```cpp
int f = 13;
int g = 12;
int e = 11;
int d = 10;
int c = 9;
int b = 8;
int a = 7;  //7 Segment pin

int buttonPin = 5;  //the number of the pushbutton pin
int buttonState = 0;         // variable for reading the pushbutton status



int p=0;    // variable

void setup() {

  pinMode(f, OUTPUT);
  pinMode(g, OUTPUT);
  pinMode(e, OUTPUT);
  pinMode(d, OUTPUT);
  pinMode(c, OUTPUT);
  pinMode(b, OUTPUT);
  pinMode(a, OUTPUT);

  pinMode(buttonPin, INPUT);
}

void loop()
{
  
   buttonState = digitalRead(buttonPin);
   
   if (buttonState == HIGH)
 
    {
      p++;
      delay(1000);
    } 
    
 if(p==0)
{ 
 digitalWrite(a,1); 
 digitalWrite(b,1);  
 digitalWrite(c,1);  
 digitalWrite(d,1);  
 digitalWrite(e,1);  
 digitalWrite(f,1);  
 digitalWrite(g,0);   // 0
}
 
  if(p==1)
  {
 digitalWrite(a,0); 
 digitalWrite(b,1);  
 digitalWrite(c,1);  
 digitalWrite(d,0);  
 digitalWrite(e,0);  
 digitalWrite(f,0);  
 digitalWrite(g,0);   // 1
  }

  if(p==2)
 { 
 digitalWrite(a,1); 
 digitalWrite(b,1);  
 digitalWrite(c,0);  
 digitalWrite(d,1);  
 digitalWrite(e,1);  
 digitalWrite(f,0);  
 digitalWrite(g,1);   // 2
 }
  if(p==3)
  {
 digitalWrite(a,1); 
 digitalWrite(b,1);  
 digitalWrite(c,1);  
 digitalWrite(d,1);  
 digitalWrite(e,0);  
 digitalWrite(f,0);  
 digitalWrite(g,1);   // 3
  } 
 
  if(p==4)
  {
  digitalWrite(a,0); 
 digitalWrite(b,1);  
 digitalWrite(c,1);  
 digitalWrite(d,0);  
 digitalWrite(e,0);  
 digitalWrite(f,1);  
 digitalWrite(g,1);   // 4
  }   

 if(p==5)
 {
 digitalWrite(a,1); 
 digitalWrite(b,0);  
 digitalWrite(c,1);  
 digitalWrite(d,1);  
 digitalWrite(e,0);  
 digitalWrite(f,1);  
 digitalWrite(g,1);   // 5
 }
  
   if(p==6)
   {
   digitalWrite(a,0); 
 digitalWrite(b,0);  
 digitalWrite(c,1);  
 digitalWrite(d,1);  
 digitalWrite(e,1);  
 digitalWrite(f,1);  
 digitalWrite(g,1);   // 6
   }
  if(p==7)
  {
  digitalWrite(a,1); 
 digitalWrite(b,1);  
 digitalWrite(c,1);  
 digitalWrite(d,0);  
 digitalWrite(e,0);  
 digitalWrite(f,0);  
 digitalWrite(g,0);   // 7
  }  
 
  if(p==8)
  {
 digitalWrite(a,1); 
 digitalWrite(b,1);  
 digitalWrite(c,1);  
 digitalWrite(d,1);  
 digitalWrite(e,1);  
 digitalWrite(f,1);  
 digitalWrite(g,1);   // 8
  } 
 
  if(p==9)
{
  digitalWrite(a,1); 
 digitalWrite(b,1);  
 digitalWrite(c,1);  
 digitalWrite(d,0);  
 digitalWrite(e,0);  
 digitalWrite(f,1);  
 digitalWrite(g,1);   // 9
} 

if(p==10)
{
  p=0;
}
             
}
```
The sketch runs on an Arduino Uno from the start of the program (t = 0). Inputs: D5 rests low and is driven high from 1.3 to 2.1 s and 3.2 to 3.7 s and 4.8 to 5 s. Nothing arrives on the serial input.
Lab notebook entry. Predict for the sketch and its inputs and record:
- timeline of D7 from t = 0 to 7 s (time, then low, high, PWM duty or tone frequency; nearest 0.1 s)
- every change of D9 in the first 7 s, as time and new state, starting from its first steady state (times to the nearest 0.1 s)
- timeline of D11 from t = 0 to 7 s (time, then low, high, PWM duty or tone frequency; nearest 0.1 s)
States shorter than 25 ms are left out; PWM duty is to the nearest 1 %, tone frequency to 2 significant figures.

0 s high; 2.3 s low; 4.2 s high
0 s high; 4.2 s low; 5.8 s high
0 s high; 2.3 s low; 4.2 s high; 5.8 s low
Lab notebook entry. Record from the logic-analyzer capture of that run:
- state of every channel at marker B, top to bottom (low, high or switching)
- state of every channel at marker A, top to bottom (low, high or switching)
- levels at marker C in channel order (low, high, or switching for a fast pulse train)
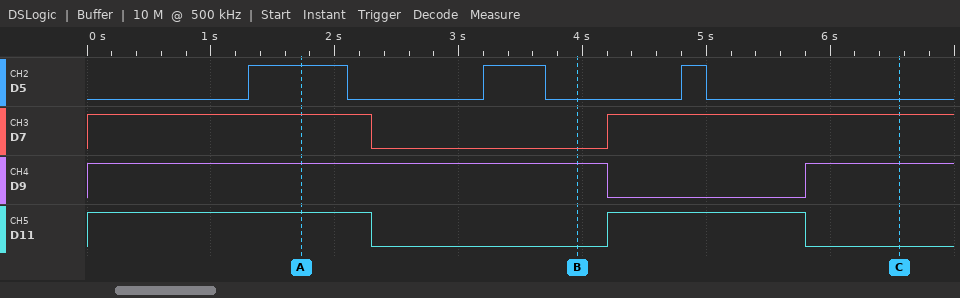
D5 low, D7 low, D9 high, D11 low
D5 high, D7 high, D9 high, D11 high
D5 low, D7 high, D9 high, D11 low
